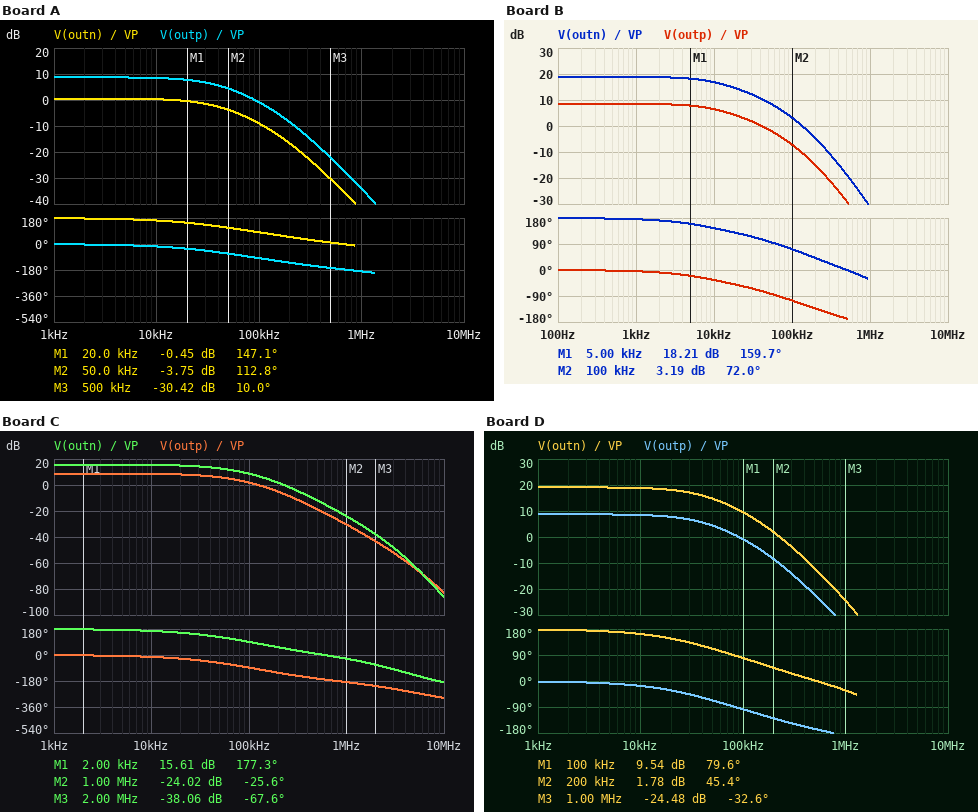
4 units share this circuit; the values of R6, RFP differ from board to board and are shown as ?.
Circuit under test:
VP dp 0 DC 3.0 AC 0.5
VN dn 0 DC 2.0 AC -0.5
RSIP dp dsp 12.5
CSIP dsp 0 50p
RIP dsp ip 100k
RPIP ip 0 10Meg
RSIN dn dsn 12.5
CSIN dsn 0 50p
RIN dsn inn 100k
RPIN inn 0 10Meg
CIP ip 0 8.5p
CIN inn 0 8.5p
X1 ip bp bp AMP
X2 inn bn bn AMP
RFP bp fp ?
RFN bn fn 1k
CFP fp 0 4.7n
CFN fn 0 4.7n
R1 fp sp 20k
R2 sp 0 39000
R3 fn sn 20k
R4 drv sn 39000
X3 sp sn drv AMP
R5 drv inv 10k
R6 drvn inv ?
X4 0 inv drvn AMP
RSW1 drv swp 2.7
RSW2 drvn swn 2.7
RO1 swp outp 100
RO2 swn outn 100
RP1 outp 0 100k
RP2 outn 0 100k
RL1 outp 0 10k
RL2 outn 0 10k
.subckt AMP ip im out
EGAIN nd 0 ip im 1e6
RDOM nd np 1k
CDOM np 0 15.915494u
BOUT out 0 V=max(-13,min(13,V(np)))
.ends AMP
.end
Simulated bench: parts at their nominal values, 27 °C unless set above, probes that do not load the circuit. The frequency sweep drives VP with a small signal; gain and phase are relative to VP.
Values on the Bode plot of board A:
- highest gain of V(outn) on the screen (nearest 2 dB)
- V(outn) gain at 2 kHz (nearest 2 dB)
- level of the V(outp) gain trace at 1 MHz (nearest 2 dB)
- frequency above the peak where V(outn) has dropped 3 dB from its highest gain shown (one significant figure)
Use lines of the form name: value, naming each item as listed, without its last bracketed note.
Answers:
highest gain of V(outn) on the screen: 0 dB
V(outn) gain at 2 kHz: 0 dB
level of the V(outp) gain trace at 1 MHz: -34 dB
frequency above the peak where V(outn) has dropped 3 dB from its highest gain shown: 40 kHz
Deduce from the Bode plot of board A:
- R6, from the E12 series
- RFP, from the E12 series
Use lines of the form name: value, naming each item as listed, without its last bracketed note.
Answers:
R6, from the E12 series: 3.9 kΩ
RFP, from the E12 series: 820 Ω
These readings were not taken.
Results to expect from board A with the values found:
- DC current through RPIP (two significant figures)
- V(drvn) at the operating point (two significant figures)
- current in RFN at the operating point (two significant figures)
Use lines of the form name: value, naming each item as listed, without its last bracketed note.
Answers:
DC current through RPIP: 300 nA
V(drvn) at the operating point: -720 mV
current in RFN at the operating point: 2.1 µA
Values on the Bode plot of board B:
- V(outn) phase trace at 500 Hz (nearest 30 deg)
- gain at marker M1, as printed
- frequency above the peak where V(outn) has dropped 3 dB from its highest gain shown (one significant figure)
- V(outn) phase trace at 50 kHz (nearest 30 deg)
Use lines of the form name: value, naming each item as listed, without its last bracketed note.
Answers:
V(outn) phase trace at 500 Hz: 180 deg
gain at marker M1, as printed: 18.21 dB
frequency above the peak where V(outn) has dropped 3 dB from its highest gain shown: 10 kHz
V(outn) phase trace at 50 kHz: 90 deg
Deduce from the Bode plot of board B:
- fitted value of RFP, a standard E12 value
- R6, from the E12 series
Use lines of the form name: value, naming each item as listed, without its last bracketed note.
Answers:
fitted value of RFP, a standard E12 value: 3.3 kΩ
R6, from the E12 series: 33 kΩ
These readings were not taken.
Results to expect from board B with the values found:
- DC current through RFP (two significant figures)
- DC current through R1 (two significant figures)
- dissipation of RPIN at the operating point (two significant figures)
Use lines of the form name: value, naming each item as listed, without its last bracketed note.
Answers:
DC current through RFP: 48 µA
DC current through R1: 48 µA
dissipation of RPIN at the operating point: 390 nW
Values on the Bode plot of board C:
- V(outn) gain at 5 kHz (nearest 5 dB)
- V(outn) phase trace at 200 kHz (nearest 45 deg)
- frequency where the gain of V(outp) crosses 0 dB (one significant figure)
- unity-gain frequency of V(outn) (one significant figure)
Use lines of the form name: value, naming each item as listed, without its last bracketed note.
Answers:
V(outn) gain at 5 kHz: 15 dB
V(outn) phase trace at 200 kHz: 45 deg
frequency where the gain of V(outp) crosses 0 dB: 100 kHz
unity-gain frequency of V(outn): 200 kHz
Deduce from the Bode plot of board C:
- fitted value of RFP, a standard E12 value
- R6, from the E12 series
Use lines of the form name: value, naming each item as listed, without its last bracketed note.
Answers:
fitted value of RFP, a standard E12 value: 470 Ω
R6, from the E12 series: 22 kΩ
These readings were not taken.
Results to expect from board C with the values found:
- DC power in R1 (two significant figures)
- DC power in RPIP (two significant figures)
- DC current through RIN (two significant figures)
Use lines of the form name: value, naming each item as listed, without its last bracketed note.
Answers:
DC power in R1: 50 µW
DC power in RPIP: 880 nW
DC current through RIN: 200 nA
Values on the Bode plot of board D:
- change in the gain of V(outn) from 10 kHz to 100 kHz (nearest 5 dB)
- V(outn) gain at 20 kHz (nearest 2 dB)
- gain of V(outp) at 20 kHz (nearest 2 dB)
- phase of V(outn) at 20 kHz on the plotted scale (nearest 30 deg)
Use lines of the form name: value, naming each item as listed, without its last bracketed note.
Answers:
change in the gain of V(outn) from 10 kHz to 100 kHz: -10 dB
V(outn) gain at 20 kHz: 18 dB
gain of V(outp) at 20 kHz: 8 dB
phase of V(outn) at 20 kHz on the plotted scale: 150 deg
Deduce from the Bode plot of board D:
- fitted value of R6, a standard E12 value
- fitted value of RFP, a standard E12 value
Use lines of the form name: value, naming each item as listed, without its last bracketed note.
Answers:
fitted value of R6, a standard E12 value: 33 kΩ
fitted value of RFP, a standard E12 value: 820 Ω
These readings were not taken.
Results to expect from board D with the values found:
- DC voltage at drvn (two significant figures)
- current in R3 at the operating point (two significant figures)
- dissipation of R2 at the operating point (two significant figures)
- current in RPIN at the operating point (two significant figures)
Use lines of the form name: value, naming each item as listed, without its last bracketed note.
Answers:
DC voltage at drvn: -6.1 V
current in R3 at the operating point: 2.1 µA
dissipation of R2 at the operating point: 96 µW
current in RPIN at the operating point: 200 nA
